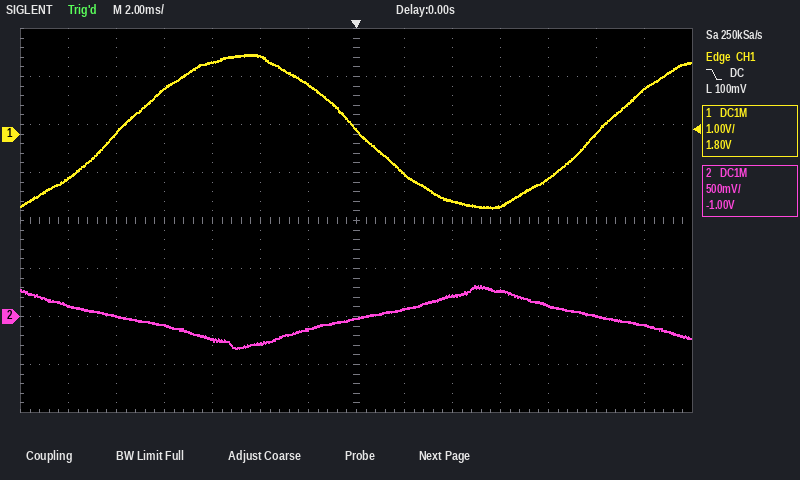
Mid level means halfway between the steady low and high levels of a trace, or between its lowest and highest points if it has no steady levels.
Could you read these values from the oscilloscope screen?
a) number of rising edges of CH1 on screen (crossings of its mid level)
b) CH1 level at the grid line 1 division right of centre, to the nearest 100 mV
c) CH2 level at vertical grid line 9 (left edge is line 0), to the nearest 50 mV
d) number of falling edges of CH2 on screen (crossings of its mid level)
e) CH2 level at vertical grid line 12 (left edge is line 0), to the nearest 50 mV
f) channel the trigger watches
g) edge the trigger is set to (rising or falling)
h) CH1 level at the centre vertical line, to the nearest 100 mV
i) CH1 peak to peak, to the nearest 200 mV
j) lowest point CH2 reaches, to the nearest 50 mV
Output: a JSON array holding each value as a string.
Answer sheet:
["2", "-800 mV", "200 mV", "2", "0 mV", "CH1", "falling", "100 mV", "3.2 V", "-350 mV"]
